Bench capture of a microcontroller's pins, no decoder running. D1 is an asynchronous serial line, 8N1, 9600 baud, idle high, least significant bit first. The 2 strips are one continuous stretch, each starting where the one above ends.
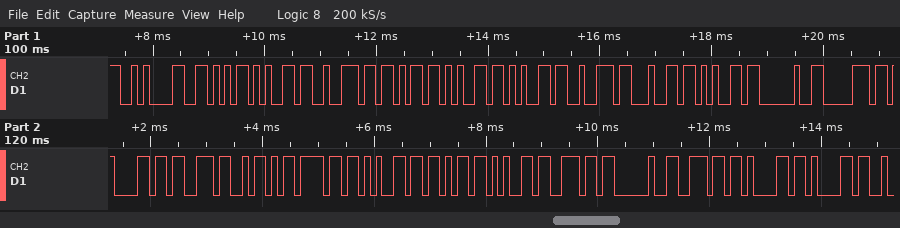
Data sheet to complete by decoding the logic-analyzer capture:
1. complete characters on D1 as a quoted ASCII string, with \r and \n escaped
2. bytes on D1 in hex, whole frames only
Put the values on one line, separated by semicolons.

"\nVerkeerde pasZoeken naa"; 0A 56 65 72 6B 65 65 72 64 65 20 70 61 73 5A 6F 65 6B 65 6E 20 6E 61 61
